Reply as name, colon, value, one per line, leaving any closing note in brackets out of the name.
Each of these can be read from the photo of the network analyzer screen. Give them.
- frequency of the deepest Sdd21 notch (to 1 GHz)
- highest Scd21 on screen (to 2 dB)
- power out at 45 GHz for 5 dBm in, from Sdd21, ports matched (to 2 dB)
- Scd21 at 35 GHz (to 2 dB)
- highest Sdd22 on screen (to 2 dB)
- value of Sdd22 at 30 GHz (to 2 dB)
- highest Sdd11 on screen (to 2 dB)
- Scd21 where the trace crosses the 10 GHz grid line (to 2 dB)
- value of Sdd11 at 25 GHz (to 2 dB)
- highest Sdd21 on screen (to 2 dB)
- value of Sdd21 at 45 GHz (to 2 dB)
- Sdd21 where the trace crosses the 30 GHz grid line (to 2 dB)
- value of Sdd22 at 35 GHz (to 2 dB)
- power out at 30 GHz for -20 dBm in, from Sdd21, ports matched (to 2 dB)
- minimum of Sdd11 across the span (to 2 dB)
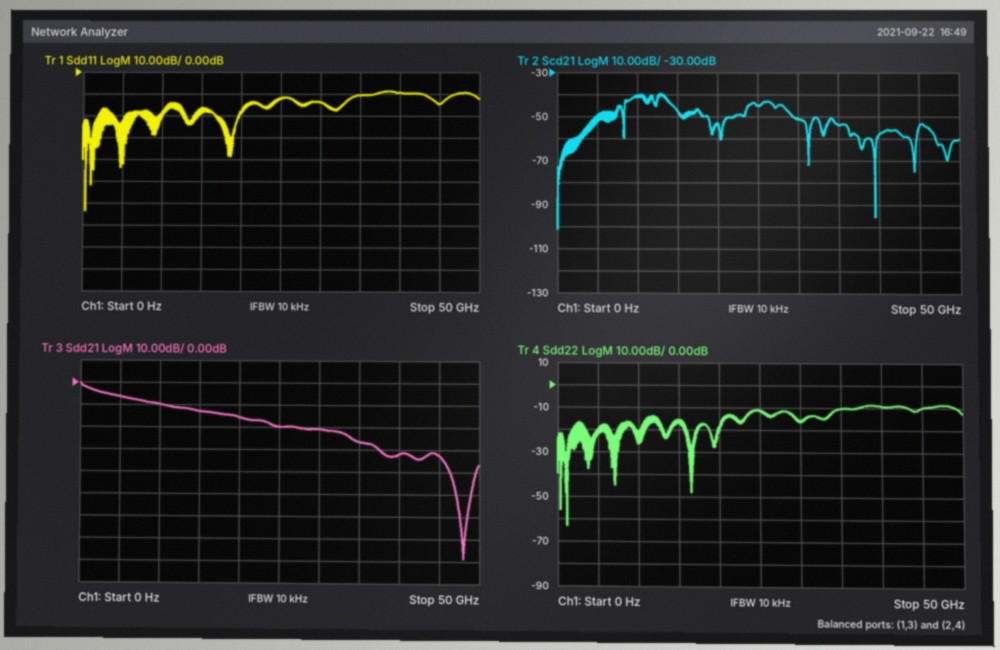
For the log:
frequency of the deepest Sdd21 notch: 48 GHz
highest Scd21 on screen: -40 dB
power out at 45 GHz for 5 dBm in, from Sdd21, ports matched: -28 dBm
Scd21 at 35 GHz: -54 dB
highest Sdd22 on screen: -8 dB
value of Sdd22 at 30 GHz: -16 dB
highest Sdd11 on screen: -8 dB
Scd21 where the trace crosses the 10 GHz grid line: -40 dB
value of Sdd11 at 25 GHz: -12 dB
highest Sdd21 on screen: 0 dB
value of Sdd21 at 45 GHz: -32 dB
Sdd21 where the trace crosses the 30 GHz grid line: -20 dB
value of Sdd22 at 35 GHz: -10 dB
power out at 30 GHz for -20 dBm in, from Sdd21, ports matched: -40 dBm
minimum of Sdd11 across the span: -64 dB
